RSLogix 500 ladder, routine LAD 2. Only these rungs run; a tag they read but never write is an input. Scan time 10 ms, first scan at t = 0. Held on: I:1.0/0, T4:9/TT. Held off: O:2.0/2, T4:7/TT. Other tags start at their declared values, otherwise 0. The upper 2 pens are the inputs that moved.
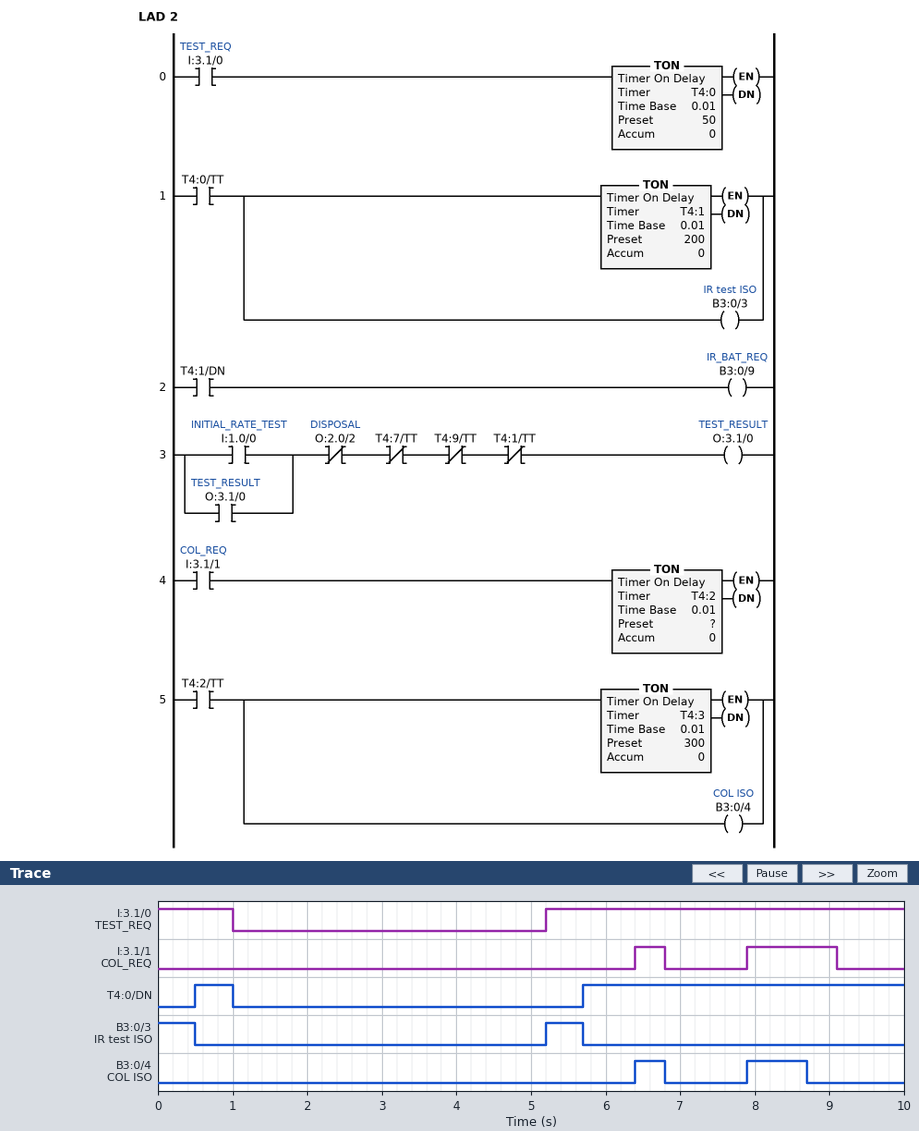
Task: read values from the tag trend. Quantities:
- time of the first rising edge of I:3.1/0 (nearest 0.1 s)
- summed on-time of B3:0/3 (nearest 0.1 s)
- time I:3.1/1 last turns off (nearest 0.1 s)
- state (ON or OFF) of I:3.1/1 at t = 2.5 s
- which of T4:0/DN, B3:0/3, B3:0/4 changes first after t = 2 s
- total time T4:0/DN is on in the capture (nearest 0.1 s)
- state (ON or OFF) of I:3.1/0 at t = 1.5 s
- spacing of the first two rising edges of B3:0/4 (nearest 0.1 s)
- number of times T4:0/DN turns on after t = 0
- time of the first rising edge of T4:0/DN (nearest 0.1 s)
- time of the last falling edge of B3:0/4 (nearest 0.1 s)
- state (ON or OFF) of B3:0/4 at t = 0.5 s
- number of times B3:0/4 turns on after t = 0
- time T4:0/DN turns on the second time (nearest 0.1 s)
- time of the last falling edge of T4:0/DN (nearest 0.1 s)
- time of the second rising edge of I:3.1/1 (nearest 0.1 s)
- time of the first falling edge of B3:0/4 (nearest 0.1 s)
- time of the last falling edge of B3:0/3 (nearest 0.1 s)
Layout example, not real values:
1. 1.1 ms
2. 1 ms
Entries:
1. 5.2 s
2. 1.0 s
3. 9.1 s
4. OFF
5. B3:0/3
6. 4.8 s
7. OFF
8. 1.5 s
9. 2
10. 0.5 s
11. 8.7 s
12. OFF
13. 2
14. 5.7 s
15. 1.0 s
16. 7.9 s
17. 6.8 s
18. 5.7 s
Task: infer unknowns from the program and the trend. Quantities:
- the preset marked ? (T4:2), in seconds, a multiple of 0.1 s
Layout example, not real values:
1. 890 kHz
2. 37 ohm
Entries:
1. 0.8 s
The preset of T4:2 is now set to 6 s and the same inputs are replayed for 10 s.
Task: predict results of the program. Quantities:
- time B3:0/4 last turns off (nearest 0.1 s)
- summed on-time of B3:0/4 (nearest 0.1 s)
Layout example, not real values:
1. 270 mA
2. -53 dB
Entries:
1. 9.1 s
2. 1.6 s
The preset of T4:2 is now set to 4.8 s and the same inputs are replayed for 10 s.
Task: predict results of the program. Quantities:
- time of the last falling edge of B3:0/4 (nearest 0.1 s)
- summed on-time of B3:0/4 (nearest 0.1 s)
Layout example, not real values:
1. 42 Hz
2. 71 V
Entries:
1. 9.1 s
2. 1.6 s
